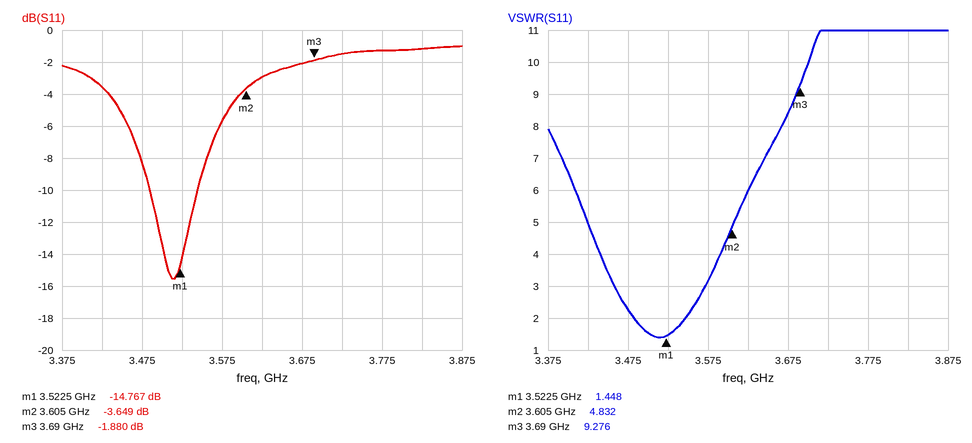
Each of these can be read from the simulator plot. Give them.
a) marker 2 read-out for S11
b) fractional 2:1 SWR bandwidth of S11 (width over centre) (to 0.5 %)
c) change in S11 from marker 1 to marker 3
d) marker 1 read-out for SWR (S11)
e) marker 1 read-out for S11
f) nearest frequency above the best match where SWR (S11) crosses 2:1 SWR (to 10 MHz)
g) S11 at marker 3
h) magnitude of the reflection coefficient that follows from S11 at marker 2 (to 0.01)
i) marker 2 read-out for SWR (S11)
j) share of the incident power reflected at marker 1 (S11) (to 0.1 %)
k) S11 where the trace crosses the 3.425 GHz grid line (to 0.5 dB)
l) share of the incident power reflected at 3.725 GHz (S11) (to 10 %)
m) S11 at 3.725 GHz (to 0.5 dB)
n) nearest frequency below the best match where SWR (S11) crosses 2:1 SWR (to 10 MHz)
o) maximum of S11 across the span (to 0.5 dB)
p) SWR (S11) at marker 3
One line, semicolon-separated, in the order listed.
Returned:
-3.649 dB; 2.0 %; 12.887 dB; 1.448; -14.767 dB; 3.55 GHz; -1.880 dB; 0.66; 4.832; 3.3 %; -3.5 dB; 70 %; -1.5 dB; 3.48 GHz; -1.0 dB; 9.276
